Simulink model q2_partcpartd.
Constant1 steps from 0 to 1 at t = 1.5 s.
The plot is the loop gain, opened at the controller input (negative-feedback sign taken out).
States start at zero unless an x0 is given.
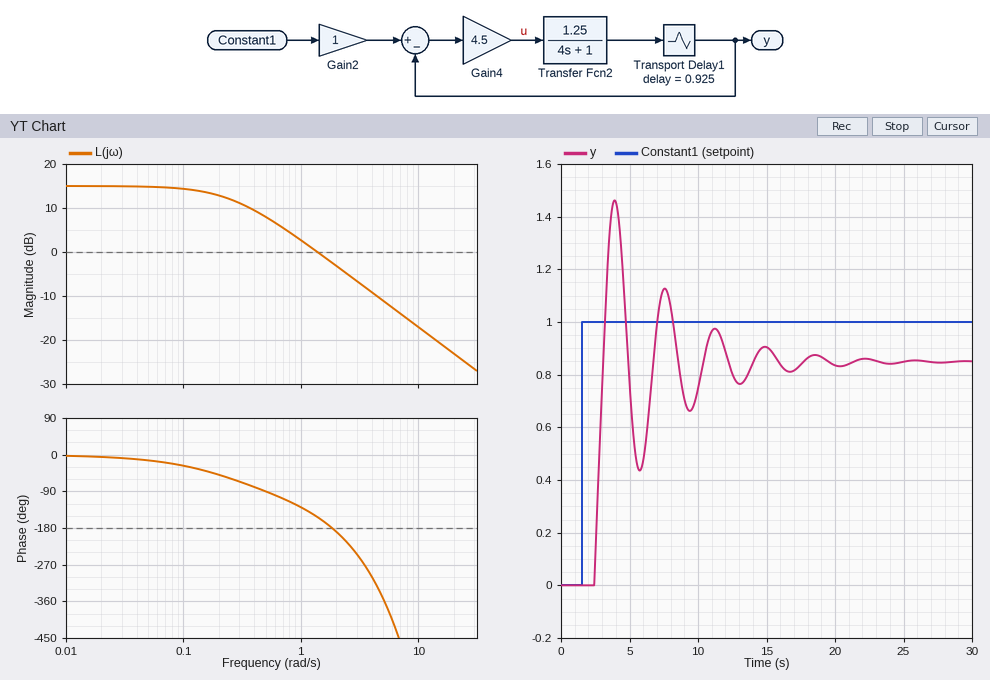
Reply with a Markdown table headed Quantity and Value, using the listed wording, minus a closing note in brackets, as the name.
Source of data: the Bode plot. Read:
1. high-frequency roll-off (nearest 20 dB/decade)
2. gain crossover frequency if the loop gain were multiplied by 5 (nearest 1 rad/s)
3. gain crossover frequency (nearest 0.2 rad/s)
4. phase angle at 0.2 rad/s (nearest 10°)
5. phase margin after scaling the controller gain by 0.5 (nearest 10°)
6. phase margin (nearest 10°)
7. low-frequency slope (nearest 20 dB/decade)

| Quantity | Value |
|---|---|
| high-frequency roll-off | -20 dB/decade |
| gain crossover frequency if the loop gain were multiplied by 5 | 7 rad/s |
| gain crossover frequency | 1.4 rad/s |
| phase angle at 0.2 rad/s | -50° |
| phase margin after scaling the controller gain by 0.5 | 80° |
| phase margin | 30° |
| low-frequency slope | 0 dB/decade |
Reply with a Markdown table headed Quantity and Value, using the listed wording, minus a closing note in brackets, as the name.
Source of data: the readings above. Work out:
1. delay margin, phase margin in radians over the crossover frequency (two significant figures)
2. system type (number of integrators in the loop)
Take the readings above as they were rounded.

| Quantity | Value |
|---|---|
| delay margin, phase margin in radians over the crossover frequency | 0.37 s |
| system type | 0 |
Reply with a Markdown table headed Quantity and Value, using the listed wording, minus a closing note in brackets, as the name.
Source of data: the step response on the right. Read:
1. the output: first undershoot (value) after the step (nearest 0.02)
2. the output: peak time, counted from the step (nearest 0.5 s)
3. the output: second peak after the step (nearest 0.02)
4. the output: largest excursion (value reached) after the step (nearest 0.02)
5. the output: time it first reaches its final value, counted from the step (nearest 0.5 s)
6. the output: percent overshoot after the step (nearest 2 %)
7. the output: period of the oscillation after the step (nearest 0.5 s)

| Quantity | Value |
|---|---|
| the output: first undershoot (value) after the step | 0.44 |
| the output: peak time, counted from the step | 2.5 s |
| the output: second peak after the step | 1.12 |
| the output: largest excursion (value reached) after the step | 1.46 |
| the output: time it first reaches its final value, counted from the step | 1.5 s |
| the output: percent overshoot after the step | 72 % |
| the output: period of the oscillation after the step | 3.5 s |
